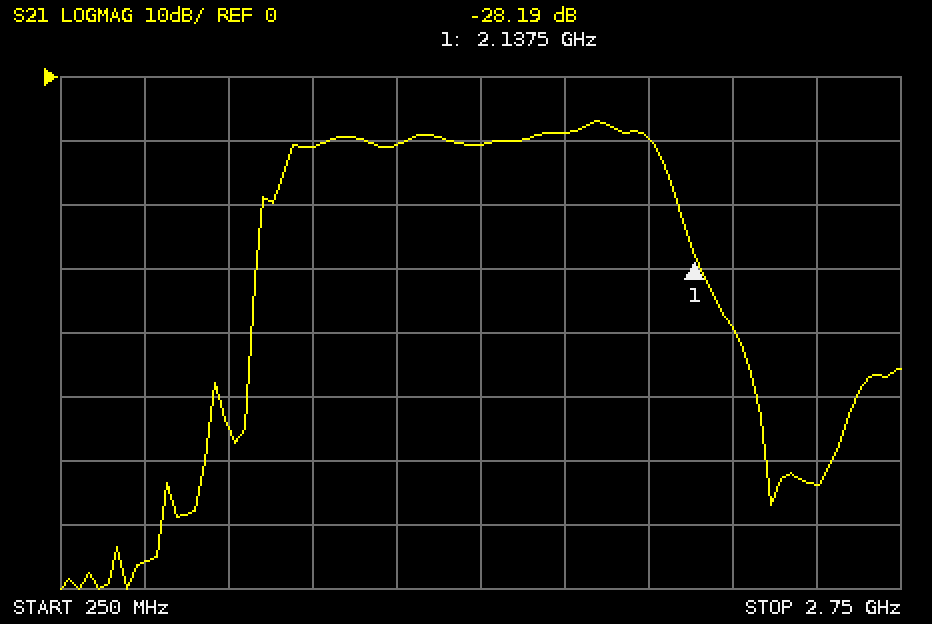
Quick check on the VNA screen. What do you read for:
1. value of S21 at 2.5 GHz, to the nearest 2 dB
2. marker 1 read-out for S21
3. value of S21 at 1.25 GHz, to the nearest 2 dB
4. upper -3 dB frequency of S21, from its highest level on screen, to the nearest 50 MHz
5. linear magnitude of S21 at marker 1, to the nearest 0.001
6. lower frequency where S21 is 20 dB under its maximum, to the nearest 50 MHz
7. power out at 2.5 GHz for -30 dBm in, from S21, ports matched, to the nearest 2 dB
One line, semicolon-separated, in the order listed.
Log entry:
-64 dB; -28.19 dB; -10 dB; 2.00 GHz; 0.039; 850 MHz; -94 dBm
